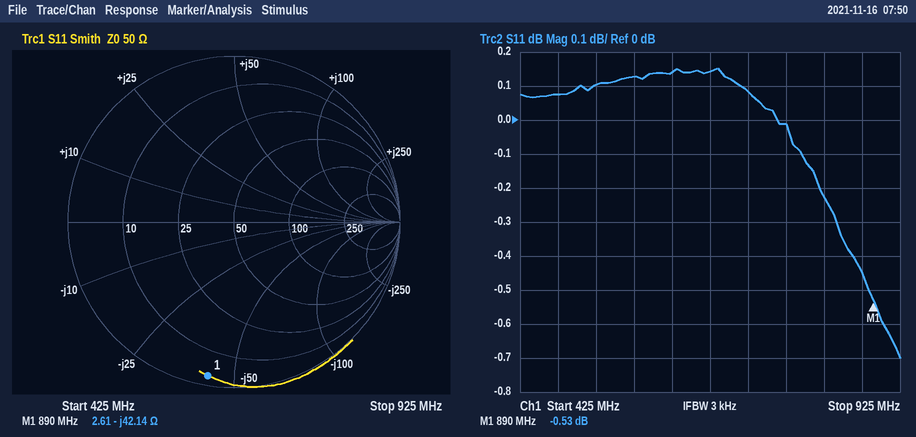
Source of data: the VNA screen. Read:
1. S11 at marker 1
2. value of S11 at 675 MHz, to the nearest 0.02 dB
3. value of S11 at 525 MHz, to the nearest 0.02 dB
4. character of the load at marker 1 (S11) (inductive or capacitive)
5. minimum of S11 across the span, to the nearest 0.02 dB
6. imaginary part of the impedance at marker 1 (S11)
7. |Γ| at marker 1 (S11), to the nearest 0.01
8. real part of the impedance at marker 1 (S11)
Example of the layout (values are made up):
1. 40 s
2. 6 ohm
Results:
1. -0.53 dB
2. 0.14 dB
3. 0.10 dB
4. capacitive
5. -0.70 dB
6. -42.14 Ω
7. 0.94
8. 2.61 Ω
